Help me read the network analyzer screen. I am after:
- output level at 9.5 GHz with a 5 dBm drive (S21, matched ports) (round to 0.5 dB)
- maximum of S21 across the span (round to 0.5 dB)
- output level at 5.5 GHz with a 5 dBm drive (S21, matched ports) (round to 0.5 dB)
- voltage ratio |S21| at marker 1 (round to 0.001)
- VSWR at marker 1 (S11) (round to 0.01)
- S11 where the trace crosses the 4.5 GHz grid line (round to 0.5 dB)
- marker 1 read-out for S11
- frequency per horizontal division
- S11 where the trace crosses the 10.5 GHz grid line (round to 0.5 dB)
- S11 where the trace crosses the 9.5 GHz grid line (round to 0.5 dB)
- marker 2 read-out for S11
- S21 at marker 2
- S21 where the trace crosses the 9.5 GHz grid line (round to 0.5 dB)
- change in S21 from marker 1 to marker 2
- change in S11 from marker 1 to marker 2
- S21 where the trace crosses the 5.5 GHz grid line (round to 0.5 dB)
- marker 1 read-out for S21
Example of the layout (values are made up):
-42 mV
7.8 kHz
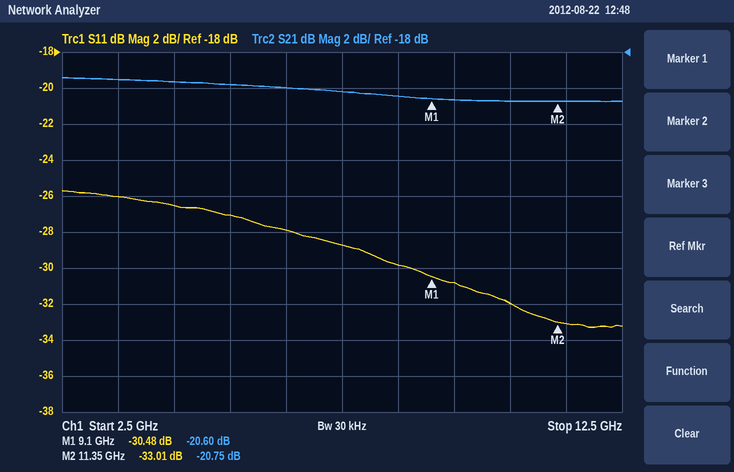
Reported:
-15.5 dBm
-19.5 dB
-15.0 dBm
0.093
1.06
-26.5 dB
-30.48 dB
1 GHz
-32.0 dB
-31.0 dB
-33.01 dB
-20.75 dB
-20.5 dB
-0.15 dB
-2.53 dB
-20.0 dB
-20.60 dB
